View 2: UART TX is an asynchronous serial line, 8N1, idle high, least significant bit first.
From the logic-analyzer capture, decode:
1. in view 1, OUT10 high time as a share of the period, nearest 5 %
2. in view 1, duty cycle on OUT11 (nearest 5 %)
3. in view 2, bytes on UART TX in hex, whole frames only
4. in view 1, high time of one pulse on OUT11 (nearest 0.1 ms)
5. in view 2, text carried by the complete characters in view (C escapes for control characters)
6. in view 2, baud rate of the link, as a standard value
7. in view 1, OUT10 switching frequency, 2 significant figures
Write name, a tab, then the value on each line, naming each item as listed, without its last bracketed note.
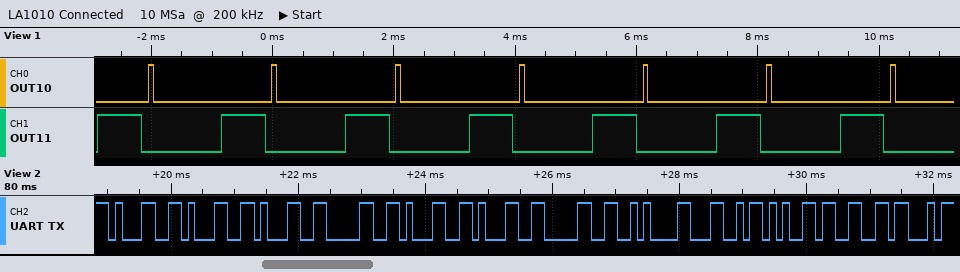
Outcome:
in view 1, OUT10 high time as a share of the period, nearest 5 %	5 %
in view 1, duty cycle on OUT11	35 %
in view 2, bytes on UART TX in hex, whole frames only	0x31 0x31 0x31 0x30 0x31 0x31 0x30 0x0A 0x4C 0x65 0x66
in view 1, high time of one pulse on OUT11	0.7 ms
in view 2, text carried by the complete characters in view	"1110110\nLef"
in view 2, baud rate of the link, as a standard value	9600 baud
in view 1, OUT10 switching frequency, 2 significant figures	490 Hz
